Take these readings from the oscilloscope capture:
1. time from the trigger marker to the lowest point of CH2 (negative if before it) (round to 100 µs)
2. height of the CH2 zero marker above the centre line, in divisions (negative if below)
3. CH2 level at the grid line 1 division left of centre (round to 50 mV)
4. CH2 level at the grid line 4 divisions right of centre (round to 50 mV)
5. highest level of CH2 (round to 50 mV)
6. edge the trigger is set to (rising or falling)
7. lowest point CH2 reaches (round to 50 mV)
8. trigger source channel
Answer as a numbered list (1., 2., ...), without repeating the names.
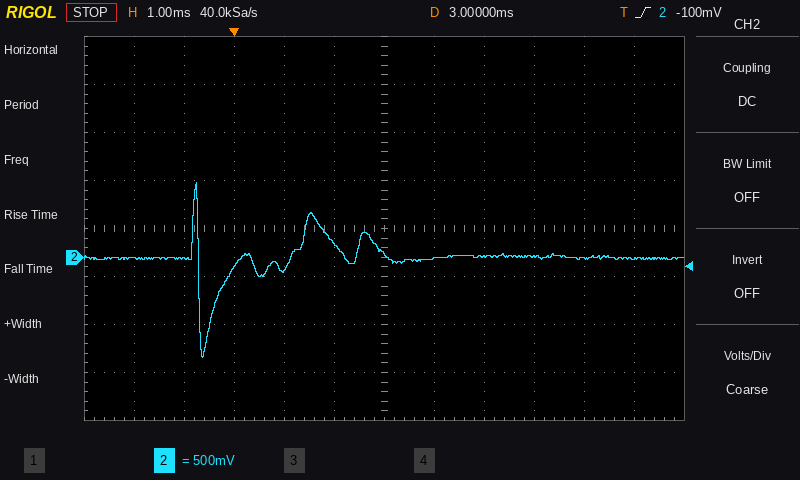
1. -600 µs
2. -0.6 div
3. 150 mV
4. 0 mV
5. 800 mV
6. rising
7. -1.05 V
8. CH2
